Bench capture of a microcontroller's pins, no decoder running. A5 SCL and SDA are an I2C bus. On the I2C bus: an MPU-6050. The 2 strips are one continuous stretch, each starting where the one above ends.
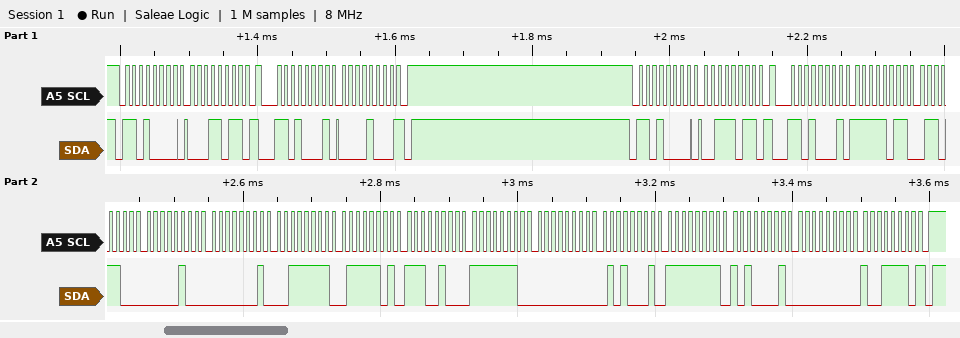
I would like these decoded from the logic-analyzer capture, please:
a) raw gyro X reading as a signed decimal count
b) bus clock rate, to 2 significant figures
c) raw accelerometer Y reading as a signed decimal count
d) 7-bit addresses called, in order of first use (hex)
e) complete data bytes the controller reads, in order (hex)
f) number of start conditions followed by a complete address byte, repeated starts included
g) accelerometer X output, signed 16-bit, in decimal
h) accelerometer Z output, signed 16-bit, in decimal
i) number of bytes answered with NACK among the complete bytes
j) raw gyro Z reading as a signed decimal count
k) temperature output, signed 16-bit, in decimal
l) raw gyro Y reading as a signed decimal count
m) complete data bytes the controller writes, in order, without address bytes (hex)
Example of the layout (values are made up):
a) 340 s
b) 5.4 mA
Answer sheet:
a) 81
b) 100 kHz
c) 1025
d) 0x68
e) 08 FB 6C 04 01 3F 7D E4 FE 00 51 FF A1 00 9E
f) 4
g) -1172
h) 16253
i) 2
j) 158
k) -6914
l) -95
m) 1B 3B
